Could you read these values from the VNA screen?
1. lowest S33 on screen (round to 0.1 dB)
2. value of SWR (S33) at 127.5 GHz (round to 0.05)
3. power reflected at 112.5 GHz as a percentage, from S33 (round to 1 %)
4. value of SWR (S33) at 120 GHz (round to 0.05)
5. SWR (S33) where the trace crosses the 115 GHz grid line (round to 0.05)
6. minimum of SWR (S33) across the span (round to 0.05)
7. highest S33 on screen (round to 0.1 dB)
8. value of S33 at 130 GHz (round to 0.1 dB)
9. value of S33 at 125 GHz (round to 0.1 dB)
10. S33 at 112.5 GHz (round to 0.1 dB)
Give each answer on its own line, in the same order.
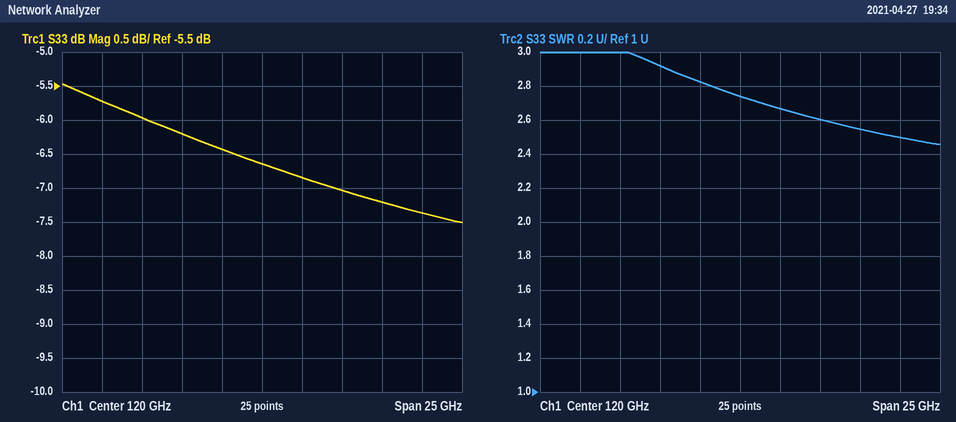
-7.5 dB
2.55
25 %
2.75
2.90
2.45
-5.5 dB
-7.4 dB
-7.0 dB
-6.0 dB
